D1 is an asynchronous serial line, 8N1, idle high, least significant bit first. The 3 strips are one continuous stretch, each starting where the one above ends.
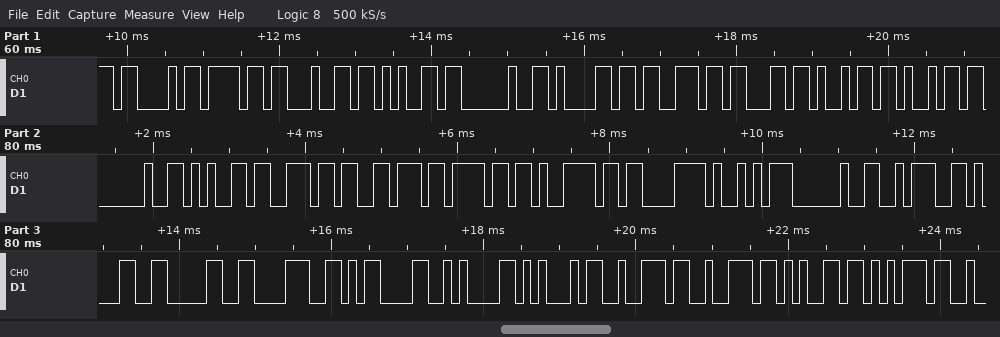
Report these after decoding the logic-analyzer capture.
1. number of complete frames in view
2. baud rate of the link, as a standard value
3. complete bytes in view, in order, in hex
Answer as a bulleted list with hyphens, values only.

- 30
- 9600 baud
- 43 6F 64 65 20 61 73 63 69 69 20 65 6E 76 6F 79 C3 A9 20 3A 31 30 38 0D 0A 45 72 72 65 75
